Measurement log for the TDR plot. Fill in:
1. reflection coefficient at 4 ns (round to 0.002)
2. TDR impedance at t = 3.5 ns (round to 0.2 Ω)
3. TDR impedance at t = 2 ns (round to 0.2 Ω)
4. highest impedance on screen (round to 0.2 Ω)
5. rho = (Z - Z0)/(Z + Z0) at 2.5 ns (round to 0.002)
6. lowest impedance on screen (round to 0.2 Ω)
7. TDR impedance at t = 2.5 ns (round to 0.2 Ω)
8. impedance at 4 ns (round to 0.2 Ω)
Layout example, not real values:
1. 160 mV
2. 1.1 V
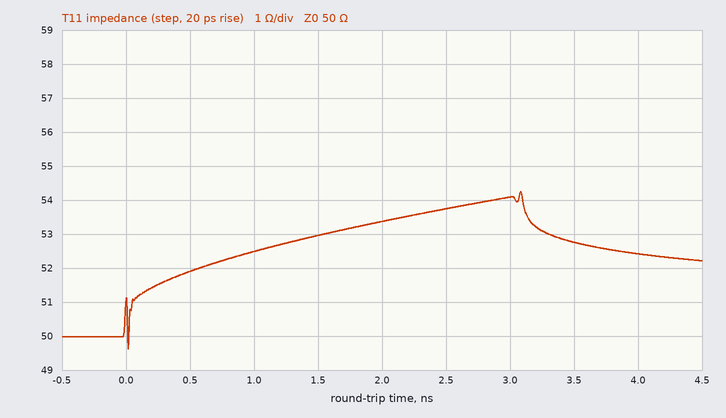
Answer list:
1. +0.024
2. 52.8 Ω
3. 53.4 Ω
4. 54.2 Ω
5. +0.036
6. 49.6 Ω
7. 53.8 Ω
8. 52.4 Ω
